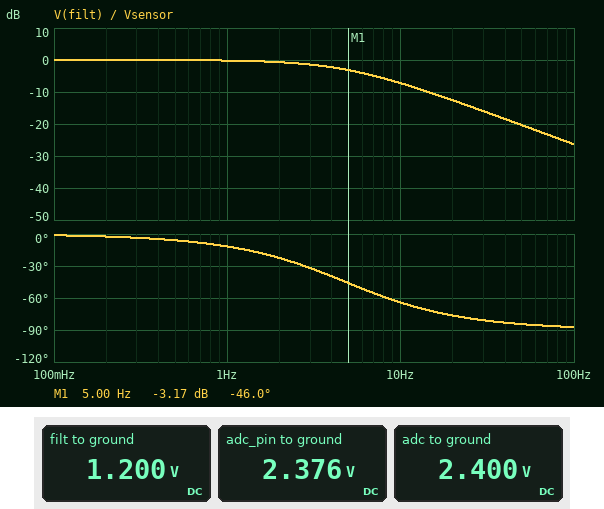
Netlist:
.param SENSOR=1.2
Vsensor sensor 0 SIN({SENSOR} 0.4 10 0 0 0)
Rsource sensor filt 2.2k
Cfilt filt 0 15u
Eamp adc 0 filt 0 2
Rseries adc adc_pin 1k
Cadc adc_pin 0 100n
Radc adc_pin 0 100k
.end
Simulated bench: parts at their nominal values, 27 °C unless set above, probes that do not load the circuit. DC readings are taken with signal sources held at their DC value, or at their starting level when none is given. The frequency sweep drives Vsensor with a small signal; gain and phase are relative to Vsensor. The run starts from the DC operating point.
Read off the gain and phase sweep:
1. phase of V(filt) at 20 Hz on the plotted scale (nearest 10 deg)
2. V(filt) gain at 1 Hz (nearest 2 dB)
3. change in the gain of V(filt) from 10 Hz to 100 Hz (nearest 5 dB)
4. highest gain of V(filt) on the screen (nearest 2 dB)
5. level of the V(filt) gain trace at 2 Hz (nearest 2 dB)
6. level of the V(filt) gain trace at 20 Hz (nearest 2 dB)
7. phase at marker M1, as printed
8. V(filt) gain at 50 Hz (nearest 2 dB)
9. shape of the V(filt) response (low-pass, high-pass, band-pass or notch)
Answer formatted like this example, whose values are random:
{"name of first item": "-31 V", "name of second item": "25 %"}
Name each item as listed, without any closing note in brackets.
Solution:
{"phase of V(filt) at 20 Hz on the plotted scale": "-80 deg", "V(filt) gain at 1 Hz": "0 dB", "change in the gain of V(filt) from 10 Hz to 100 Hz": "-20 dB", "highest gain of V(filt) on the screen": "0 dB", "level of the V(filt) gain trace at 2 Hz": "0 dB", "level of the V(filt) gain trace at 20 Hz": "-12 dB", "phase at marker M1, as printed": "-46.0 deg", "V(filt) gain at 50 Hz": "-20 dB", "shape of the V(filt) response": "low-pass"}
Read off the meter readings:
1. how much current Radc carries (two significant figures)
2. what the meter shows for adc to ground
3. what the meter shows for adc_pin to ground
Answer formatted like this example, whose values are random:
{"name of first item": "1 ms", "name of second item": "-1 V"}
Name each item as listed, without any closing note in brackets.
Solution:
{"how much current Radc carries": "24 µA", "what the meter shows for adc to ground": "2.400 V", "what the meter shows for adc_pin to ground": "2.376 V"}
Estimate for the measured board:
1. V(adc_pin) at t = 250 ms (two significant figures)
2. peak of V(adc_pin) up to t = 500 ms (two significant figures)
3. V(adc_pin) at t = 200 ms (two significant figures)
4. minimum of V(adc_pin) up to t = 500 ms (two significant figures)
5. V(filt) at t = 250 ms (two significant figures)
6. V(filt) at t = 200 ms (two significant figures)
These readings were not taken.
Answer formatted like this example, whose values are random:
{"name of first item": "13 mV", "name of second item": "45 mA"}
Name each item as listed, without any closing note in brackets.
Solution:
{"V(adc_pin) at t = 250 ms": "2.7 V", "peak of V(adc_pin) up to t = 500 ms": "2.8 V", "V(adc_pin) at t = 200 ms": "2.1 V", "minimum of V(adc_pin) up to t = 500 ms": "2.0 V", "V(filt) at t = 250 ms": "1.4 V", "V(filt) at t = 200 ms": "1.0 V"}
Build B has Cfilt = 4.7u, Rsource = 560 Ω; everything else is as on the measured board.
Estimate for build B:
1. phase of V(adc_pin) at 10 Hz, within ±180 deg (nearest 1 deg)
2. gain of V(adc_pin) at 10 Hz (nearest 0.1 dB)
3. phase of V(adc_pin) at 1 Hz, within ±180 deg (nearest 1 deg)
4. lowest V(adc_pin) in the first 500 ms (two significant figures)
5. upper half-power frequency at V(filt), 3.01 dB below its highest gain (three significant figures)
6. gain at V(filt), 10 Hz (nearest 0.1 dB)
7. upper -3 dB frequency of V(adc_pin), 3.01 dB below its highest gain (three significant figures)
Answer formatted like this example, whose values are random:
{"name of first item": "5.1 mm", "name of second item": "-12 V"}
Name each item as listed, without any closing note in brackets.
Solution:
{"phase of V(adc_pin) at 10 Hz, within ±180 deg": "-10 deg", "gain of V(adc_pin) at 10 Hz": "5.8 dB", "phase of V(adc_pin) at 1 Hz, within ±180 deg": "-1 deg", "lowest V(adc_pin) in the first 500 ms": "1.6 V", "upper half-power frequency at V(filt), 3.01 dB below its highest gain": "60.5 Hz", "gain at V(filt), 10 Hz": "-0.1 dB", "upper -3 dB frequency of V(adc_pin), 3.01 dB below its highest gain": "60.4 Hz"}
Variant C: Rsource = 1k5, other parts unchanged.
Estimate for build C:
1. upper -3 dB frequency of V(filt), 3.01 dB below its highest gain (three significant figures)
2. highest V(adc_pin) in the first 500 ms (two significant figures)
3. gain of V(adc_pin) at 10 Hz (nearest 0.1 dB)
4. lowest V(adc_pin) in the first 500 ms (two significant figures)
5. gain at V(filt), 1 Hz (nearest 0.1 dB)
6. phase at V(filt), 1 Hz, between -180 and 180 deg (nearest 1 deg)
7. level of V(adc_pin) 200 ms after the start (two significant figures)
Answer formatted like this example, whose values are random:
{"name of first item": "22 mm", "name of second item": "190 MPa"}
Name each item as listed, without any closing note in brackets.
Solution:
{"upper -3 dB frequency of V(filt), 3.01 dB below its highest gain": "7.07 Hz", "highest V(adc_pin) in the first 500 ms": "2.9 V", "gain of V(adc_pin) at 10 Hz": "1.2 dB", "lowest V(adc_pin) in the first 500 ms": "1.9 V", "gain at V(filt), 1 Hz": "-0.1 dB", "phase at V(filt), 1 Hz, between -180 and 180 deg": "-8 deg", "level of V(adc_pin) 200 ms after the start": "2.0 V"}
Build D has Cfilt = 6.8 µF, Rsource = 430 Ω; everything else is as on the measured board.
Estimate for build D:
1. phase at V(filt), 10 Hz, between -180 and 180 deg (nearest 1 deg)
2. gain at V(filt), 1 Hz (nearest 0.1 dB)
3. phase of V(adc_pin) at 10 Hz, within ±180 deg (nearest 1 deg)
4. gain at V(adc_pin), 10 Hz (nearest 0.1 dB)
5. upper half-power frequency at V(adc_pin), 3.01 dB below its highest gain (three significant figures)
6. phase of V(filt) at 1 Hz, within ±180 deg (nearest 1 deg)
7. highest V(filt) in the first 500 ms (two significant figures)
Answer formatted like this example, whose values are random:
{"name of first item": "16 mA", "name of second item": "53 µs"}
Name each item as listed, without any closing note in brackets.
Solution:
{"phase at V(filt), 10 Hz, between -180 and 180 deg": "-10 deg", "gain at V(filt), 1 Hz": "0 dB", "phase of V(adc_pin) at 10 Hz, within ±180 deg": "-11 deg", "gain at V(adc_pin), 10 Hz": "5.8 dB", "upper half-power frequency at V(adc_pin), 3.01 dB below its highest gain": "54.4 Hz", "phase of V(filt) at 1 Hz, within ±180 deg": "-1 deg", "highest V(filt) in the first 500 ms": "1.6 V"}
